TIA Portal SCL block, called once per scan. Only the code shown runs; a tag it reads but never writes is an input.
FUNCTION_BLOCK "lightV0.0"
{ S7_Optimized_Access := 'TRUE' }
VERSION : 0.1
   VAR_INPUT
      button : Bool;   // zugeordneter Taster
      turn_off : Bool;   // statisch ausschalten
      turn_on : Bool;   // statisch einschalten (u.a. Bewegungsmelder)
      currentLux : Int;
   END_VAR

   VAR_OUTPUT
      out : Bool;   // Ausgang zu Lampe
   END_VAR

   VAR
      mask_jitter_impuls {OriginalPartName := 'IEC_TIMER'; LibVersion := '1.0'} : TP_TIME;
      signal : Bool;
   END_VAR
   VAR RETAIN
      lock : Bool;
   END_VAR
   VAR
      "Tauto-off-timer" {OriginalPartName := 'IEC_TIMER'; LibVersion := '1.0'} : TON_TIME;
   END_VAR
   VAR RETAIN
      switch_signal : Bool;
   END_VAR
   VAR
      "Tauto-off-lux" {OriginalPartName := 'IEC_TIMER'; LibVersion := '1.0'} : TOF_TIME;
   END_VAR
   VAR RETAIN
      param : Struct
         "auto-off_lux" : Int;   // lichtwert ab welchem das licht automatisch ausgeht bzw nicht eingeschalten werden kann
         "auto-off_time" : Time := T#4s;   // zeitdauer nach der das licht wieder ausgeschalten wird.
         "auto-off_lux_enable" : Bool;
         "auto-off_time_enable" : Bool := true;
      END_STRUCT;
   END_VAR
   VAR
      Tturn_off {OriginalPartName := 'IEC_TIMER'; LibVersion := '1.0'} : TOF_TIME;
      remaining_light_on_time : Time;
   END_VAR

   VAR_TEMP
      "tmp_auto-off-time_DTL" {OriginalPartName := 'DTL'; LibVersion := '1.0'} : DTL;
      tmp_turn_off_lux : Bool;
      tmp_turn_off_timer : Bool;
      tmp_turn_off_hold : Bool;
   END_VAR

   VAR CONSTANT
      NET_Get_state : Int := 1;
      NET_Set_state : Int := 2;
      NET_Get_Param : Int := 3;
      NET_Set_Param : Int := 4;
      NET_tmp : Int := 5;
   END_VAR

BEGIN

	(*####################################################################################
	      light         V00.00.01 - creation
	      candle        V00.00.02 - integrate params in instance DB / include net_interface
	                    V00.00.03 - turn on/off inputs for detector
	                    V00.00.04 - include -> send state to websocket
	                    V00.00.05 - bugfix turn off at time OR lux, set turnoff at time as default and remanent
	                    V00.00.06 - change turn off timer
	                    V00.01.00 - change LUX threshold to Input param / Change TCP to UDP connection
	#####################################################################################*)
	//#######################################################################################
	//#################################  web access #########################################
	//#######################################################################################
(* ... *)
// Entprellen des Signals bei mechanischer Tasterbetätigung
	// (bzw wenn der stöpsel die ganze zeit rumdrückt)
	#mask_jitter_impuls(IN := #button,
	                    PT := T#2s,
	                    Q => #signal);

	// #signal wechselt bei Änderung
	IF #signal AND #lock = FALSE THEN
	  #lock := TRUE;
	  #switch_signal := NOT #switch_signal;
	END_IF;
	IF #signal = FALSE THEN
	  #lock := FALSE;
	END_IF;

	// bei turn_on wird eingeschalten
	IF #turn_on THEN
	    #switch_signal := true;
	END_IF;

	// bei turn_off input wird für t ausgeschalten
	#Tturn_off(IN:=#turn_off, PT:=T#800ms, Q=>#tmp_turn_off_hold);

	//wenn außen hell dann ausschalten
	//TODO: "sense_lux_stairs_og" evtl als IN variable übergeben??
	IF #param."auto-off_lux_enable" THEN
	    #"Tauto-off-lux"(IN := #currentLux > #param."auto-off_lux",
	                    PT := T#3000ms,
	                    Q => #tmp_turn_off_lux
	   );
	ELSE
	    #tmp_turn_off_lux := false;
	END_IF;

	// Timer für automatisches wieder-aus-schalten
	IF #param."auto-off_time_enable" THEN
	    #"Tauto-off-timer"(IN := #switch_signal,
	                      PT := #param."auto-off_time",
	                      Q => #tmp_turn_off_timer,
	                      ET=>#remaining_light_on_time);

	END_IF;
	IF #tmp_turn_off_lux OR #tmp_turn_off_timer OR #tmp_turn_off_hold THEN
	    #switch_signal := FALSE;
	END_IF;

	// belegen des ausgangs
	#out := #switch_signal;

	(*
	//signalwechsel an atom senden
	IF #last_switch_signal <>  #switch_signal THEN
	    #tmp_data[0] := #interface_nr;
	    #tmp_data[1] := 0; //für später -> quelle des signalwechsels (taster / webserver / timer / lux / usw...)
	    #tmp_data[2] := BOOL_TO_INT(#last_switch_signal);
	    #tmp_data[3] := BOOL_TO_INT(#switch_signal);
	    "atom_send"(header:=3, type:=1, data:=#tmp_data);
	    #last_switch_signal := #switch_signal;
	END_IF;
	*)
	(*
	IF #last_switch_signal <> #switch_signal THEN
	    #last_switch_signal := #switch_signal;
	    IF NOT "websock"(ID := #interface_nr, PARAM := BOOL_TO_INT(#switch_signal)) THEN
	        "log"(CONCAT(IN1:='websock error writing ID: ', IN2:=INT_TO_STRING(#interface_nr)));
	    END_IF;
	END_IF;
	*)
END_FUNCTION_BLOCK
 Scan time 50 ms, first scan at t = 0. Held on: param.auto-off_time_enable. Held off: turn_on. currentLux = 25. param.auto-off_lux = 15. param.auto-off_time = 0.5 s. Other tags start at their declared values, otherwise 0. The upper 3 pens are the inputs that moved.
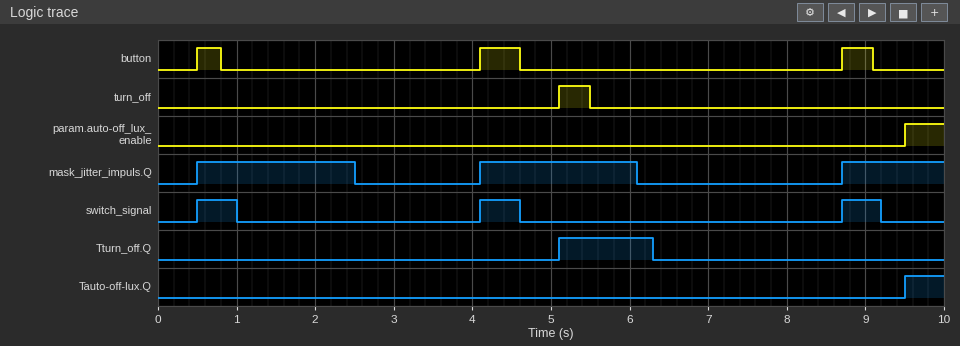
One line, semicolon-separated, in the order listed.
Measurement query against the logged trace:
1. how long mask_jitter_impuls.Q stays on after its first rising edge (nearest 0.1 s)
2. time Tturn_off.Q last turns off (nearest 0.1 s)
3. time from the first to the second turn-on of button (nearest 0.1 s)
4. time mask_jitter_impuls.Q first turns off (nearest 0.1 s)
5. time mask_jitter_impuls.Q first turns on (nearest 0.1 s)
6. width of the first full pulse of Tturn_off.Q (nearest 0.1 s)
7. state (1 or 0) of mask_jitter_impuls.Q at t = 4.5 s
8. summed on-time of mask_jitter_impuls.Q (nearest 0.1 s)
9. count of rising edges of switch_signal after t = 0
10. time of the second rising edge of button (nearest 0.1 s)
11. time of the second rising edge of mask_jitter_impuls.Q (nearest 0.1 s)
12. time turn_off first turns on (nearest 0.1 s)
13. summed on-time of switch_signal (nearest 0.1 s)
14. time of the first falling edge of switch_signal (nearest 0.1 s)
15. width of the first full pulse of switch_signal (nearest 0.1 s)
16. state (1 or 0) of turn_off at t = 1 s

2.0 s; 6.3 s; 3.6 s; 2.5 s; 0.5 s; 1.2 s; 1; 5.3 s; 3; 4.1 s; 4.1 s; 5.1 s; 1.5 s; 1.0 s; 0.5 s; 0
